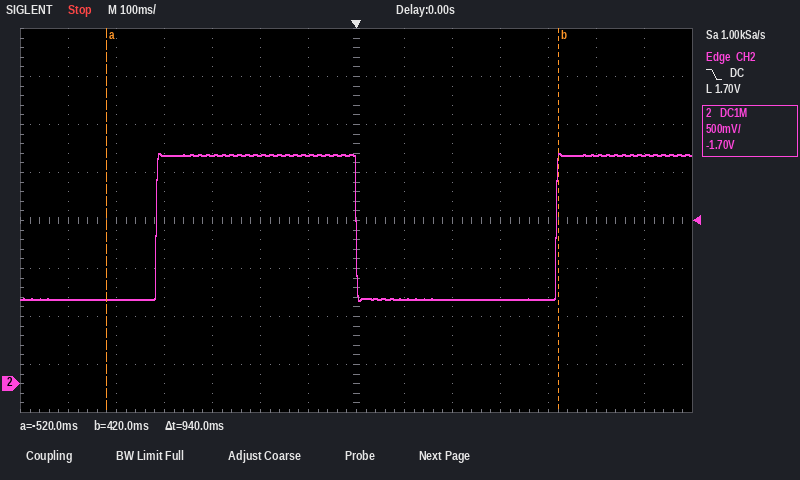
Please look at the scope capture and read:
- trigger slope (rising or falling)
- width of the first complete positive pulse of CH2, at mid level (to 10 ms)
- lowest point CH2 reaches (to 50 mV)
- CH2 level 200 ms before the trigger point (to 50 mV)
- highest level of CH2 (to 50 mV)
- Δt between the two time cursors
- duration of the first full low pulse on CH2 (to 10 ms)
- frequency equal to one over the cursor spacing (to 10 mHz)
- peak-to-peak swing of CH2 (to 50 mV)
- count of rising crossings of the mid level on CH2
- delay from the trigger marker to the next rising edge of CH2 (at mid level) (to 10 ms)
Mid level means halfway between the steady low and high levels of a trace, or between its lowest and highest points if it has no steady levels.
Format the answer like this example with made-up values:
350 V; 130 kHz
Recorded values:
falling; 420 ms; 850 mV; 2.40 V; 2.40 V; 940 ms; 420 ms; 1.06 Hz; 1.55 V; 2; 420 ms
